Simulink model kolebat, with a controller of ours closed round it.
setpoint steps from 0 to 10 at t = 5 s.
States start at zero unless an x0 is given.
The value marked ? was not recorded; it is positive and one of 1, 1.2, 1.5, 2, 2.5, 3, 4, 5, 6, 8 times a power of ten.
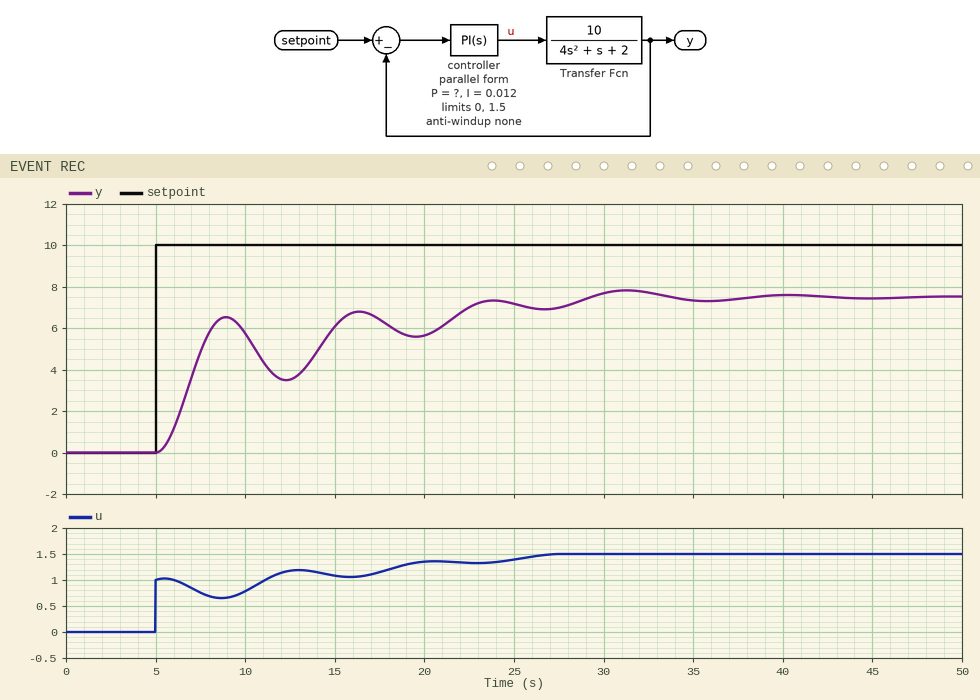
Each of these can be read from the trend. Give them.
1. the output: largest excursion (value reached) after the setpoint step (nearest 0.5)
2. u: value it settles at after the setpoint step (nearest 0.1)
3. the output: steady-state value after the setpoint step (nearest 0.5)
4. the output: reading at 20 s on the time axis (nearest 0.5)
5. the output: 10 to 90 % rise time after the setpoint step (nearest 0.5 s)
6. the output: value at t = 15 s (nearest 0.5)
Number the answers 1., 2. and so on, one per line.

1. 8.0
2. 1.5
3. 7.5
4. 5.5
5. 10.0 s
6. 6.0
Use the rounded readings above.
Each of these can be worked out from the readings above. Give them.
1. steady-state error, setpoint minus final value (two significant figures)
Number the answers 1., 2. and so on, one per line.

1. 2.5
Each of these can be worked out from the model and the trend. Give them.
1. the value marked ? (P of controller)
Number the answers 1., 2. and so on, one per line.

1. 0.1
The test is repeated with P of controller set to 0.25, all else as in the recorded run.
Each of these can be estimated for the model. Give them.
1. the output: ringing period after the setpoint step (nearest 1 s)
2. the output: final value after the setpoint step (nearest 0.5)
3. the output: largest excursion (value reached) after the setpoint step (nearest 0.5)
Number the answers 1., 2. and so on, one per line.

1. 7 s
2. 7.5
3. 9.0
